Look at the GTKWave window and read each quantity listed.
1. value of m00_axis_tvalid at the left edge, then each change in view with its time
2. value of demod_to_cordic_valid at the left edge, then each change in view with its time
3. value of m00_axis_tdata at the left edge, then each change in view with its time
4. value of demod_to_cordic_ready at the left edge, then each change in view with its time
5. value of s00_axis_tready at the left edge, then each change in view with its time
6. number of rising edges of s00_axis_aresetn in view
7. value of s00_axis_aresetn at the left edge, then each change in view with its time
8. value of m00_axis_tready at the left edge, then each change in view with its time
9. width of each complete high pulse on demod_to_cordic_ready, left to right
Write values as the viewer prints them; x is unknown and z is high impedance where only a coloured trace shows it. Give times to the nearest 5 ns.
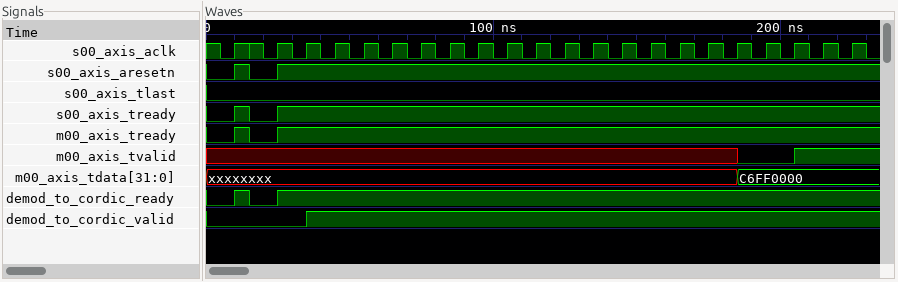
x, 0 at 185 ns, 1 at 205 ns
0, 1 at 35 ns
xxxxxxxx, C6FF0000 at 185 ns
0, 1 at 10 ns, 0 at 15 ns, 1 at 25 ns
0, 1 at 10 ns, 0 at 15 ns, 1 at 25 ns
2
0, 1 at 10 ns, 0 at 15 ns, 1 at 25 ns
0, 1 at 10 ns, 0 at 15 ns, 1 at 25 ns
5 ns
